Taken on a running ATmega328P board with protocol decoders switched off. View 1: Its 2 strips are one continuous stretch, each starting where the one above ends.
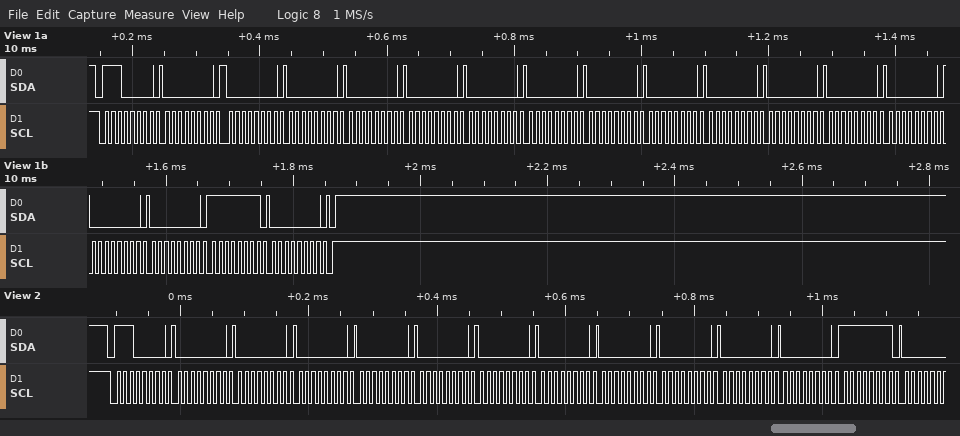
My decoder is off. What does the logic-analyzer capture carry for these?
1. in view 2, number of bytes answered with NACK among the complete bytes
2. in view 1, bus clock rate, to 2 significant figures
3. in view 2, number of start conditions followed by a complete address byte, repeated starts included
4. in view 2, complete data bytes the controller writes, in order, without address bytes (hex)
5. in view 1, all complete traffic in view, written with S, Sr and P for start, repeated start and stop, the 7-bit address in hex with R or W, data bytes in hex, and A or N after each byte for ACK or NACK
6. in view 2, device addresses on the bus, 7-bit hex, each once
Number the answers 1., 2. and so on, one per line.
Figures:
1. 0
2. 100 kHz
3. 1
4. 00 00 00 00 00 00 00 00 00 00 00 FF
5. S 70W A 00 A 00 A 00 A 00 A 00 A 00 A 00 A 00 A 00 A 00 A 00 A 00 A 00 A 00 A 00 A FF A 00 A P
6. 0x70
